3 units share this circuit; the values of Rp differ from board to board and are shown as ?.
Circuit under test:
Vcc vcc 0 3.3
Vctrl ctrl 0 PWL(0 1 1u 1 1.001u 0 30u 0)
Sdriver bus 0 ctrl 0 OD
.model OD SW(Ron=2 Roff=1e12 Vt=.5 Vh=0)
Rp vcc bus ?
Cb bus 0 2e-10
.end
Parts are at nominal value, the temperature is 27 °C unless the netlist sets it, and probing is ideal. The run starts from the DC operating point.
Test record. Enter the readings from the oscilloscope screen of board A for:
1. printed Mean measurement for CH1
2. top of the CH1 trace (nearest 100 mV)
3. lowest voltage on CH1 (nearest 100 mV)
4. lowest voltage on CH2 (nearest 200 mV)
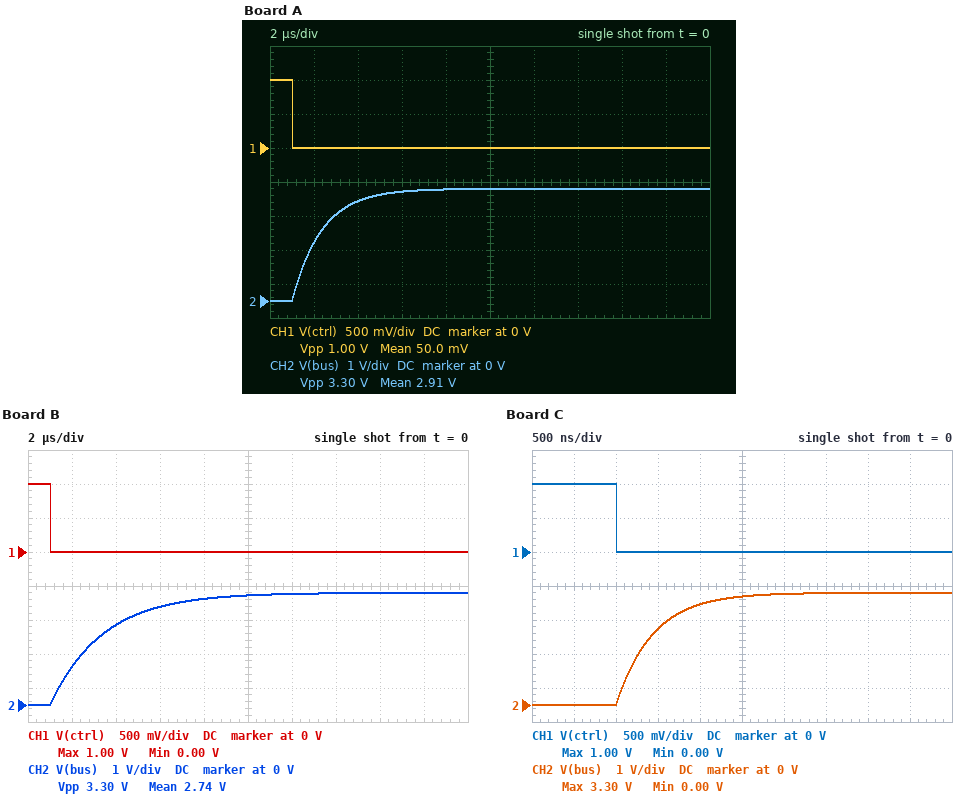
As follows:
50.0 mV
1.0 V
0 V
0 V
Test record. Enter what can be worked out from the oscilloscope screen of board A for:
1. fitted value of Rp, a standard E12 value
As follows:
6.8 kΩ
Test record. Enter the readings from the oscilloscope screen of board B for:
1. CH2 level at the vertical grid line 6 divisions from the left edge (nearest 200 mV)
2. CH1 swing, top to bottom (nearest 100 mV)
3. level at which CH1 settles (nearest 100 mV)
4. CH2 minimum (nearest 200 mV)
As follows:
3.2 V
1.0 V
0 V
0 V
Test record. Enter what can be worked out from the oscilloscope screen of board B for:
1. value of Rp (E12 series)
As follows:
12 kΩ
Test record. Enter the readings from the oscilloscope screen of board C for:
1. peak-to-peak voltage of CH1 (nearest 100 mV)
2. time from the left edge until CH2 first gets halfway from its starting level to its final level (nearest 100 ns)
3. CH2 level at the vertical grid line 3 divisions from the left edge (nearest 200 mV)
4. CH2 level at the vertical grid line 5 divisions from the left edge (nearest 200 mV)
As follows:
1.0 V
1.3 µs
2.2 V
3.2 V
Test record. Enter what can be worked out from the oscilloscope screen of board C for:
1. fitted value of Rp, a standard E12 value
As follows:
2.2 kΩ
